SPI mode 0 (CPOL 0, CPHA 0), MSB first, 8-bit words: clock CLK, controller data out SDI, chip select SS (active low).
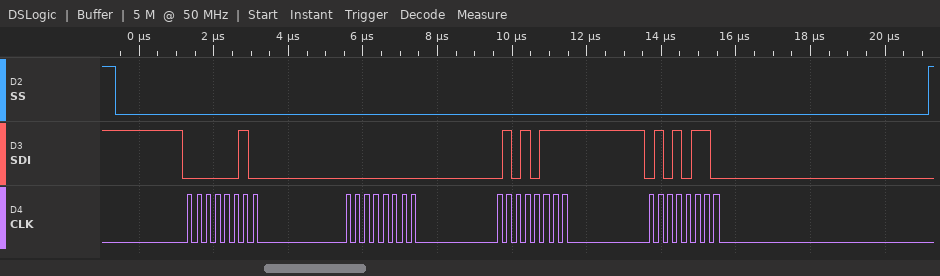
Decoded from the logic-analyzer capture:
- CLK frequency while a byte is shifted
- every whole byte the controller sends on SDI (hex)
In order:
4 MHz
02 00 57 56
